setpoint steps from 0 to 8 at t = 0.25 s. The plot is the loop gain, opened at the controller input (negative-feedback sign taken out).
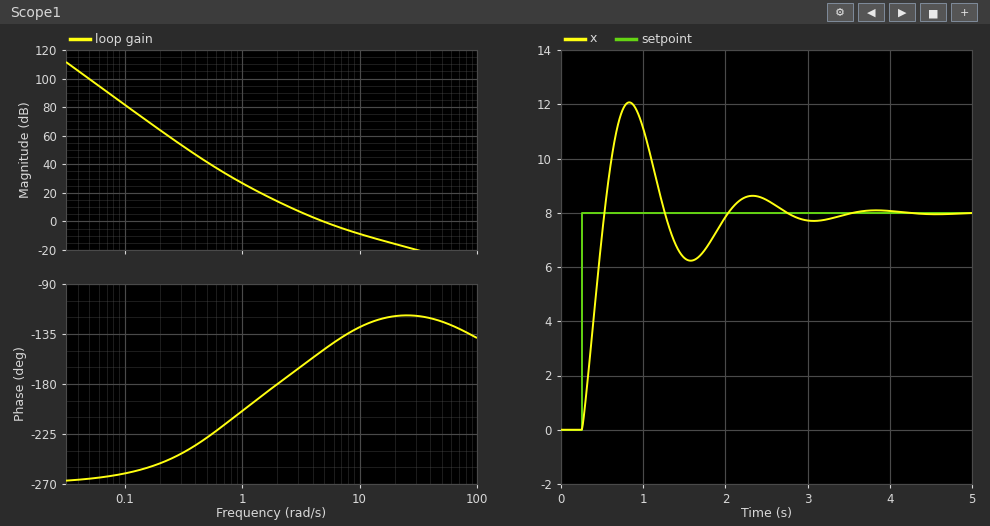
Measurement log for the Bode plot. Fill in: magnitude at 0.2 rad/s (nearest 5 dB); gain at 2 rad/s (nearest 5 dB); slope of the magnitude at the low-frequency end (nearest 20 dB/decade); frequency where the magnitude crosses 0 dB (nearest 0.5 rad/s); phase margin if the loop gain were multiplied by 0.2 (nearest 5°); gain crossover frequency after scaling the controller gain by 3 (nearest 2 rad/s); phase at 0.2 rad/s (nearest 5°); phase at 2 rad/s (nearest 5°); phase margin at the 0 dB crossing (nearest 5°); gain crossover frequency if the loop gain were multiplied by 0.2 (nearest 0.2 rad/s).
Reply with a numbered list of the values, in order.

1. 65 dB
2. 15 dB
3. -60 dB/decade
4. 5.0 rad/s
5. 0°
6. 10 rad/s
7. -250°
8. -180°
9. 30°
10. 2.0 rad/s
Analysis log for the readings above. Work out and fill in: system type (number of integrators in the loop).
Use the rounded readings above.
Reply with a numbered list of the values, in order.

1. 3
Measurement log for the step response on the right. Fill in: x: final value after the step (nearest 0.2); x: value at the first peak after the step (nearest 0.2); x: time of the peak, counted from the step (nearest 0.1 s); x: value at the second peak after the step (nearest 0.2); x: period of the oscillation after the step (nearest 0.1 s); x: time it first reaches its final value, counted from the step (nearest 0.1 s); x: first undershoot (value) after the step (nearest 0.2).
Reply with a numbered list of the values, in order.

1. 8.0
2. 12.0
3. 0.6 s
4. 8.6
5. 1.5 s
6. 0.3 s
7. 6.2
